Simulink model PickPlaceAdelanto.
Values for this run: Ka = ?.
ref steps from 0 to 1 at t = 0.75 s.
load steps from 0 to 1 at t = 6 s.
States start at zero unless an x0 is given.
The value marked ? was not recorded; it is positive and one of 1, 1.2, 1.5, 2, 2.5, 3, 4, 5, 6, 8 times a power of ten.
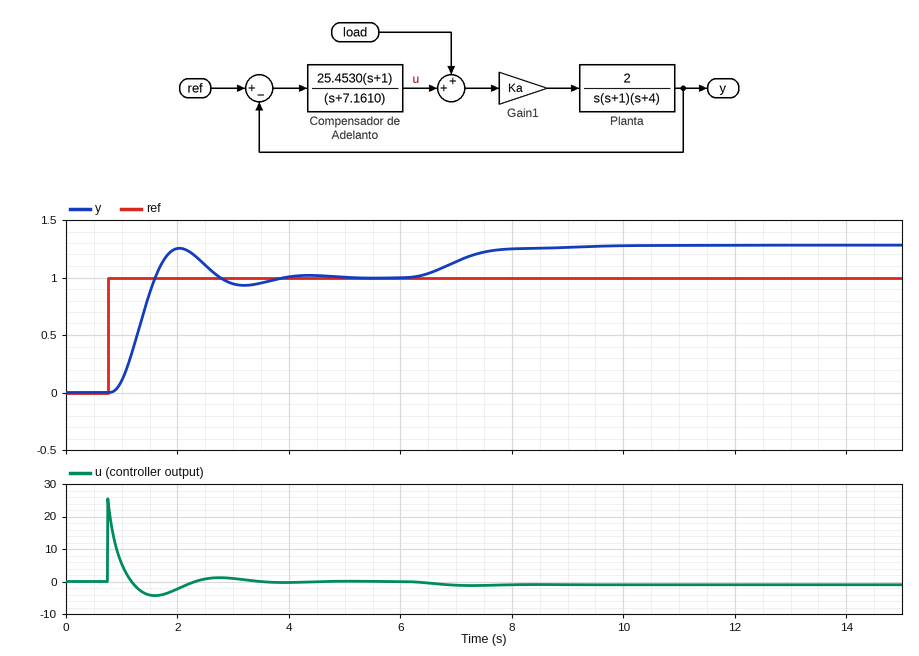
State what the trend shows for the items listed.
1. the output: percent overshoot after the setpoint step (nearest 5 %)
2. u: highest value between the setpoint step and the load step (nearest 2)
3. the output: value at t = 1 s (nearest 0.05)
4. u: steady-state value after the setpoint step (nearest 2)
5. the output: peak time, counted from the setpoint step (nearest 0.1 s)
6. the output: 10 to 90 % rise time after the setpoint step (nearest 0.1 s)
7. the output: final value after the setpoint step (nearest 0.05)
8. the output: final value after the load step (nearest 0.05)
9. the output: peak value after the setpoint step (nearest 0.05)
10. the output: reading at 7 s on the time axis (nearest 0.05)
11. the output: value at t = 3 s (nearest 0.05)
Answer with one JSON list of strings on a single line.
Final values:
["25 %", "26", "0.10", "0", "1.3 s", "0.5 s", "1.00", "1.30", "1.25", "1.15", "0.95"]
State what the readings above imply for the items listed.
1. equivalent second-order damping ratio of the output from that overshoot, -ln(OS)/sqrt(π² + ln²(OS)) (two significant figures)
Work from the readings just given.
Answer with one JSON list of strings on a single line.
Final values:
["0.40"]
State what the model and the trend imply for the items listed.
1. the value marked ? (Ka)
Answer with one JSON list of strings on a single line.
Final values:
["1.5"]
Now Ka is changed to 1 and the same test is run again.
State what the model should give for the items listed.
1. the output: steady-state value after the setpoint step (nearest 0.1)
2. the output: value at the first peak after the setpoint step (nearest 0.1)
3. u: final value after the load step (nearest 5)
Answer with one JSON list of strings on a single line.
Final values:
["1.0", "1.1", "0"]
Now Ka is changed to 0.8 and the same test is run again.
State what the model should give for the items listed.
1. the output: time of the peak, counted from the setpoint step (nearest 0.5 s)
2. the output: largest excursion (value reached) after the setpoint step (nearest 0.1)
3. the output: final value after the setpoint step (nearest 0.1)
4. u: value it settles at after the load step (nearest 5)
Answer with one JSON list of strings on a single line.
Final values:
["2.0 s", "1.1", "1.0", "0"]
